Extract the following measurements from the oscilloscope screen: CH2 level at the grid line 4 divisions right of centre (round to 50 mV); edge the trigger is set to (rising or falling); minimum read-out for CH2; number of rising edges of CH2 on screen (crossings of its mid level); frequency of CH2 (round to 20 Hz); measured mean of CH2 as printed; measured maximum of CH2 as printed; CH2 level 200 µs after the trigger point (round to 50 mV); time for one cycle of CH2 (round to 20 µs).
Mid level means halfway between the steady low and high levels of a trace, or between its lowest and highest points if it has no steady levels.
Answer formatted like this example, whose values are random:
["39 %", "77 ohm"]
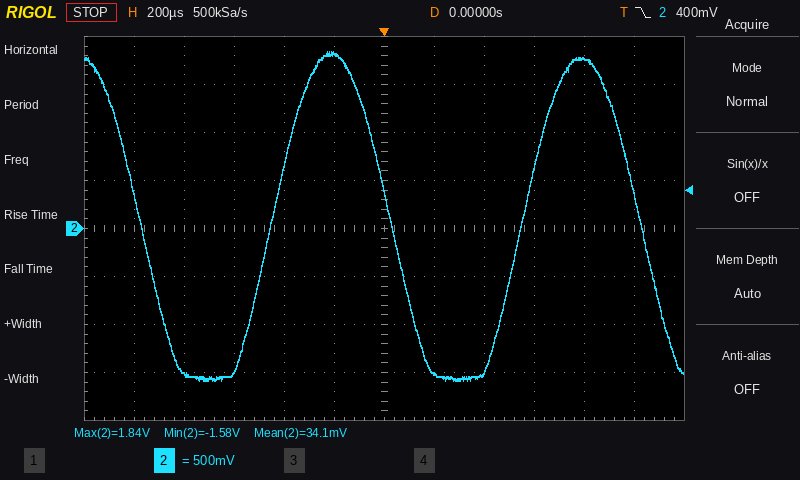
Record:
["1.75 V", "falling", "-1.58 V", "2", "1.00 kHz", "34.1 mV", "1.84 V", "-1.50 V", "1.00 ms"]
